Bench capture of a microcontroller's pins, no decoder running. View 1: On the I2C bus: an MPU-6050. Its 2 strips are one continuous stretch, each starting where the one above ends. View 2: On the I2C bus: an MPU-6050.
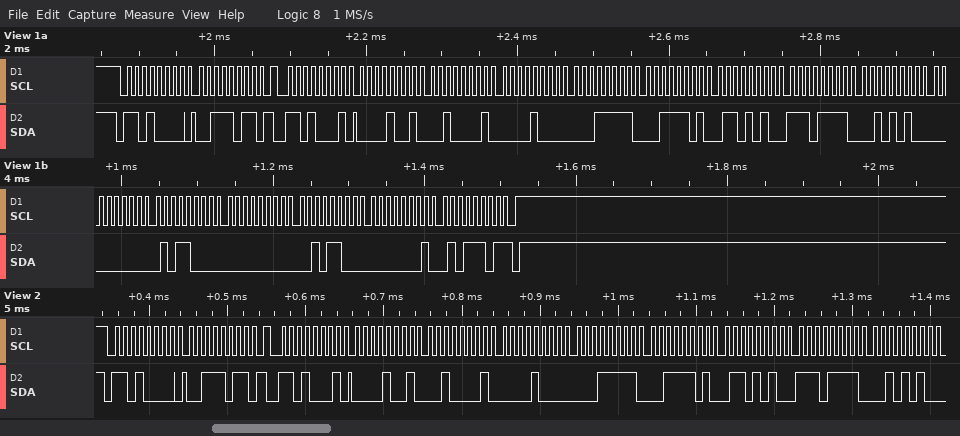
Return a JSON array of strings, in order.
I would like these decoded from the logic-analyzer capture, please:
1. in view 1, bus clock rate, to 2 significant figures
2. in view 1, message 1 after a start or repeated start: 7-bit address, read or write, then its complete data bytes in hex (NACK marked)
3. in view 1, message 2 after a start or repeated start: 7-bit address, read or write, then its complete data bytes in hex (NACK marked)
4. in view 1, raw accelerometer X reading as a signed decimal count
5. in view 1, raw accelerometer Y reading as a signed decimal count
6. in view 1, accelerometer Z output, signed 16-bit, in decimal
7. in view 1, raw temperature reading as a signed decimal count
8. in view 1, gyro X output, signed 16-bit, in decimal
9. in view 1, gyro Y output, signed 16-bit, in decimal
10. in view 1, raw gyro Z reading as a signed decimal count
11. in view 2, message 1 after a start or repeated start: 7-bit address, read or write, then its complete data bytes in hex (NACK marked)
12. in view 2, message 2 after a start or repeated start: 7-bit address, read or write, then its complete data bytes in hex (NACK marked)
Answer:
["100 kHz", "0x68 write: 3B", "0x68 read: 09 21 08 1F 3D 6A EF 2A 00 58 00 2C 01 5D NACK", "2337", "2079", "15722", "-4310", "88", "44", "349", "0x68 write: 3B", "0x68 read: 09 21 08 1F 3D 6A EF 2A"]
